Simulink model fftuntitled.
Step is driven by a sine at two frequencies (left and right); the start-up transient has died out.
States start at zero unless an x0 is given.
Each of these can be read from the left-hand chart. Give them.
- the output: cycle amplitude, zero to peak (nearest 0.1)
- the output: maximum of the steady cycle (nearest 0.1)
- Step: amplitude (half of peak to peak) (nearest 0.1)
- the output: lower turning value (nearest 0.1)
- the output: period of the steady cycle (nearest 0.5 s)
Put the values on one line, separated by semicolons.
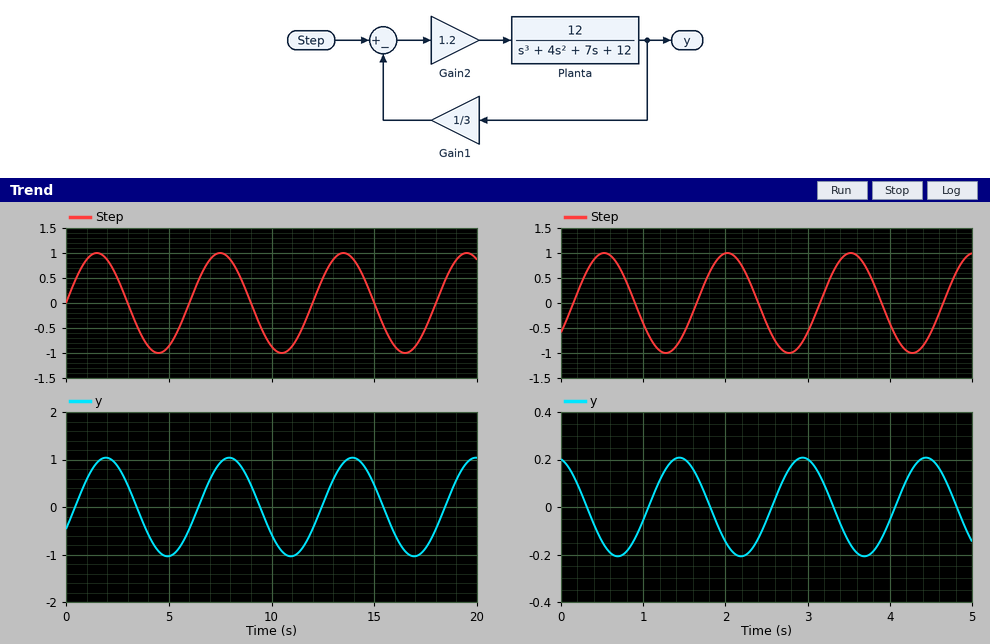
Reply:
1.0; 1.0; 1.0; -1.0; 6.0 s
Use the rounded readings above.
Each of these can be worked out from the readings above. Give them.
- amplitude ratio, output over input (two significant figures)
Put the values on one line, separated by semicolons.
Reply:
1.0
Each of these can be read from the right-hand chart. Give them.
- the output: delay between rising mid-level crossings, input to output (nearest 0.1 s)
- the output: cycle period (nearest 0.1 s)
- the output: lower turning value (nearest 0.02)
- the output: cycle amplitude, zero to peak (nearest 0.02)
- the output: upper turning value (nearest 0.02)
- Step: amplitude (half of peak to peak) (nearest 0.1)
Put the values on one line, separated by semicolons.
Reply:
0.9 s; 1.5 s; -0.20; 0.20; 0.20; 1.0
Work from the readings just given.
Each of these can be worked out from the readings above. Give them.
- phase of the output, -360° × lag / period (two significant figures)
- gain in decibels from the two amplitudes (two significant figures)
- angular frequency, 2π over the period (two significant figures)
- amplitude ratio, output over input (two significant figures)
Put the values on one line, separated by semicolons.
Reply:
-220°; -14 dB; 4.2 rad/s; 0.20
